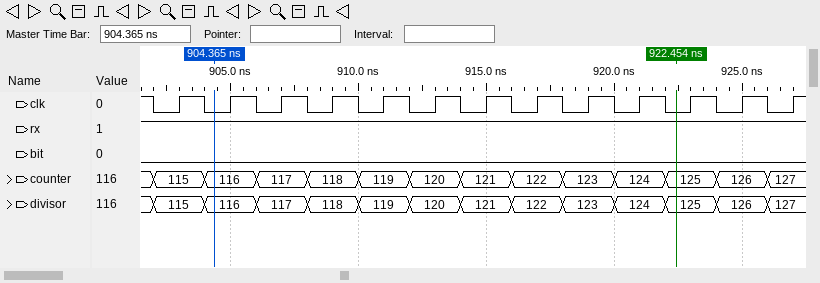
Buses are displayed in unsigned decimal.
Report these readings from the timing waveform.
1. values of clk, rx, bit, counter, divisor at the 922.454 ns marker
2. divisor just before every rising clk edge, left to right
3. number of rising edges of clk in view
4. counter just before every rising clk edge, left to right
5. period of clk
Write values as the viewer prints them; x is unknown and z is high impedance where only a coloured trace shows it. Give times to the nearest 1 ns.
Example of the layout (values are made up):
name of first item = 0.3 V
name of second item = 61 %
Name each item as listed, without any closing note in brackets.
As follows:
values of clk, rx, bit, counter, divisor at the 922.454 ns marker = clk=0, rx=1, bit=0, counter=125, divisor=125
divisor just before every rising clk edge, left to right = 115, 116, 117, 118, 119, 120, 121, 122, 123, 124, 125, 126, 127
number of rising edges of clk in view = 13
counter just before every rising clk edge, left to right = 115, 116, 117, 118, 119, 120, 121, 122, 123, 124, 125, 126, 127
period of clk = 2 ns
